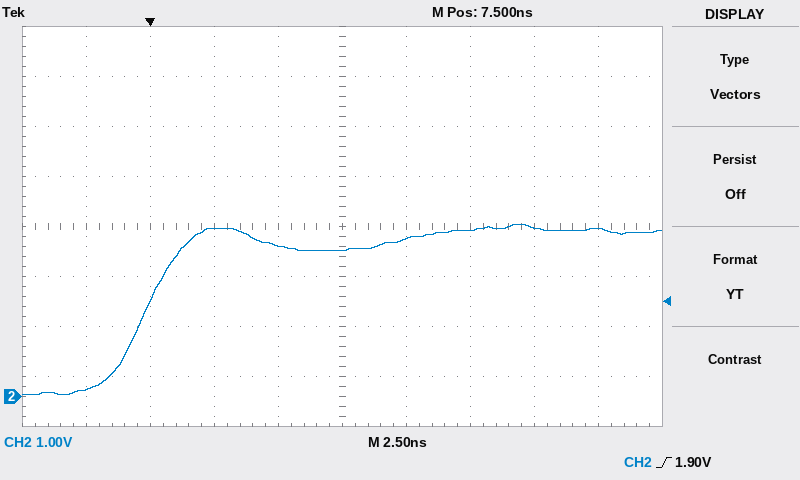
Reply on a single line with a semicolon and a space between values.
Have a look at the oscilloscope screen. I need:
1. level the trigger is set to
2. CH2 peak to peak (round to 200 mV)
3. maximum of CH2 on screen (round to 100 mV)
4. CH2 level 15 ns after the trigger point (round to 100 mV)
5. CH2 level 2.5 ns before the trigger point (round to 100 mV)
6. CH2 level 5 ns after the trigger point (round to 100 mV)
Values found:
1.90 V; 3.4 V; 3.4 V; 3.4 V; 100 mV; 3.0 V
